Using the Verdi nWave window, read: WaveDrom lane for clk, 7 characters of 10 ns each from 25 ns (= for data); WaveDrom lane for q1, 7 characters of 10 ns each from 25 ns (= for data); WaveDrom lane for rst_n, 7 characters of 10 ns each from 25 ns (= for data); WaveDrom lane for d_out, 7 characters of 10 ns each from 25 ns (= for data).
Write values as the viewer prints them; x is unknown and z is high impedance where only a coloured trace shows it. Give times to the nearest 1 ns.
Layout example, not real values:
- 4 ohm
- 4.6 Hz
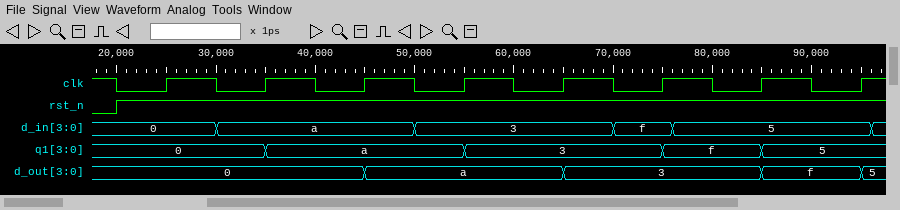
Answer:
- {name: 'clk', wave: 'p......'}
- {name: 'q1', wave: '==.=.==', data: '0 a 3 f 5'}
- {name: 'rst_n', wave: '1......'}
- {name: 'd_out', wave: '=.=.=.=', data: '0 a 3 f'}
